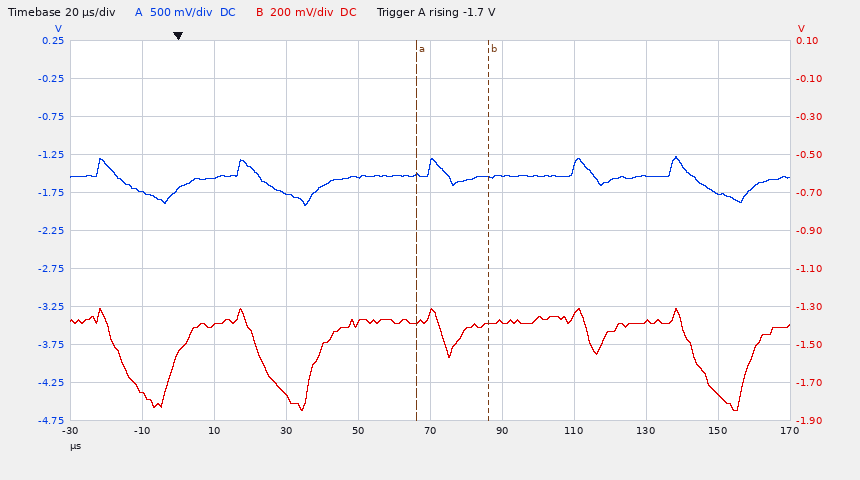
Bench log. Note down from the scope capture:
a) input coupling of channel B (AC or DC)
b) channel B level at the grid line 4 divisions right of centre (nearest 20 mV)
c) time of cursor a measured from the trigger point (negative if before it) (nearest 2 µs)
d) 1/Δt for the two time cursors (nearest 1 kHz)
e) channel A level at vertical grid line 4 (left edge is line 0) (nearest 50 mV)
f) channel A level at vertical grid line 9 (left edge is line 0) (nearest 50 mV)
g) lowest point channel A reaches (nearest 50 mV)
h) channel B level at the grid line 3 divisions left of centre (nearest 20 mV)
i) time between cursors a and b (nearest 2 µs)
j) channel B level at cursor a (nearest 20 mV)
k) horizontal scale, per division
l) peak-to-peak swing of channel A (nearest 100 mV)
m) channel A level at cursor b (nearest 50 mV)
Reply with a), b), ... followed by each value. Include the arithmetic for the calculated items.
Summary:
a) DC
b) -1.76 V
c) +66 µs
d) 1 / 20 µs ≈ 50 kHz
e) -1.55 V
f) -1.75 V
g) -1.90 V
h) -1.40 V
i) 20 µs
j) -1.38 V
k) 20 µs
l) 600 mV
m) -1.55 V
